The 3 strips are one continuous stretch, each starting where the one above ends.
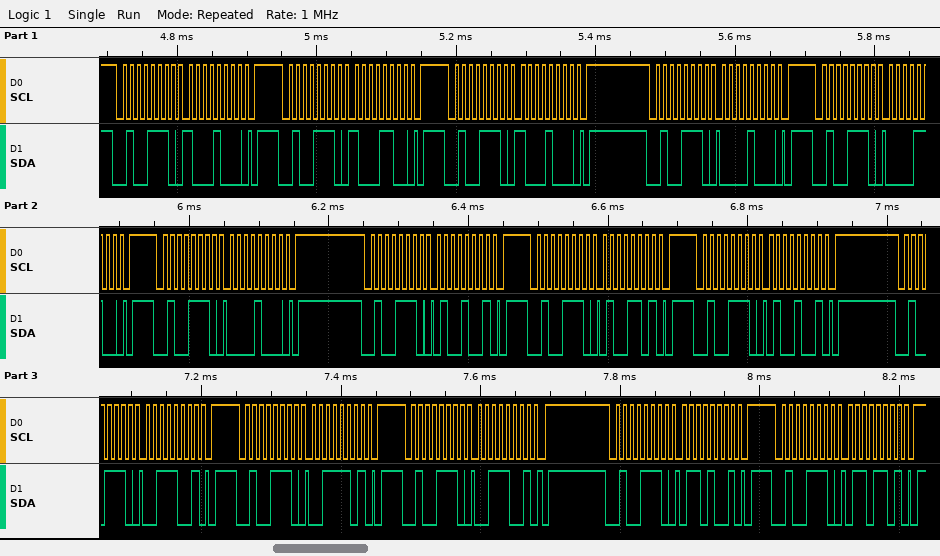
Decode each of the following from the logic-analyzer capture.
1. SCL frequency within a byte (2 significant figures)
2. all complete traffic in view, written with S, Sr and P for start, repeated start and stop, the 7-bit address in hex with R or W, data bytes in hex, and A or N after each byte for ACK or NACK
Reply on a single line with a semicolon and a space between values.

100 kHz; S 27W A 88 A P S 27W A 8C A P S 27W A 88 A P S 27W A 08 A P S 27W A 0C A P S 27W A 08 A P S 27W A 49 A P S 27W A 4D A P S 27W A 49 A P S 27W A 39 A P S 27W A 3D A P S 27W A 39 A P S 27W A 69 A P S 27W A 6D A P
